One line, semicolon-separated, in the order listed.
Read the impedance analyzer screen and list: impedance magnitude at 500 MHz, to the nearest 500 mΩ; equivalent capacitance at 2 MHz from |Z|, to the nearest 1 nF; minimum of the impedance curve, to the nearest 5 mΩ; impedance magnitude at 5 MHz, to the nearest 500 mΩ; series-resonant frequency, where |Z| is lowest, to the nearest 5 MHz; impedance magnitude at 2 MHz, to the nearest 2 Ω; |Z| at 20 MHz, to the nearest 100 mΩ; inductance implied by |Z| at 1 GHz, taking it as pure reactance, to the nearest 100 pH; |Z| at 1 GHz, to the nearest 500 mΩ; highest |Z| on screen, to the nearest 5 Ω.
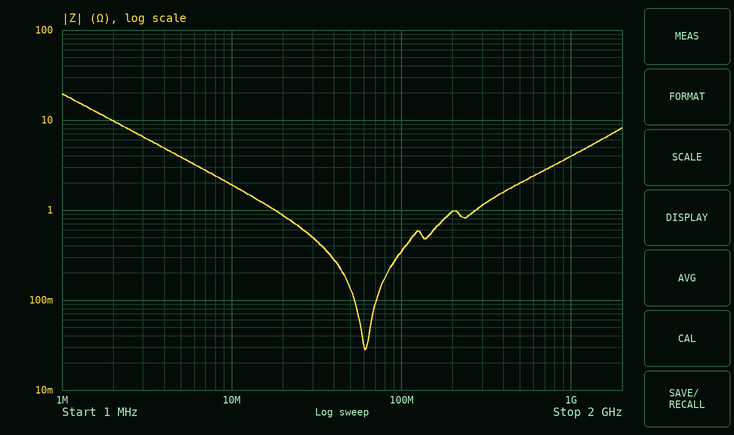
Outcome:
2.0 Ω; 8 nF; 30 mΩ; 4.0 Ω; 60 MHz; 10 Ω; 900 mΩ; 600 pH; 4.0 Ω; 20 Ω
